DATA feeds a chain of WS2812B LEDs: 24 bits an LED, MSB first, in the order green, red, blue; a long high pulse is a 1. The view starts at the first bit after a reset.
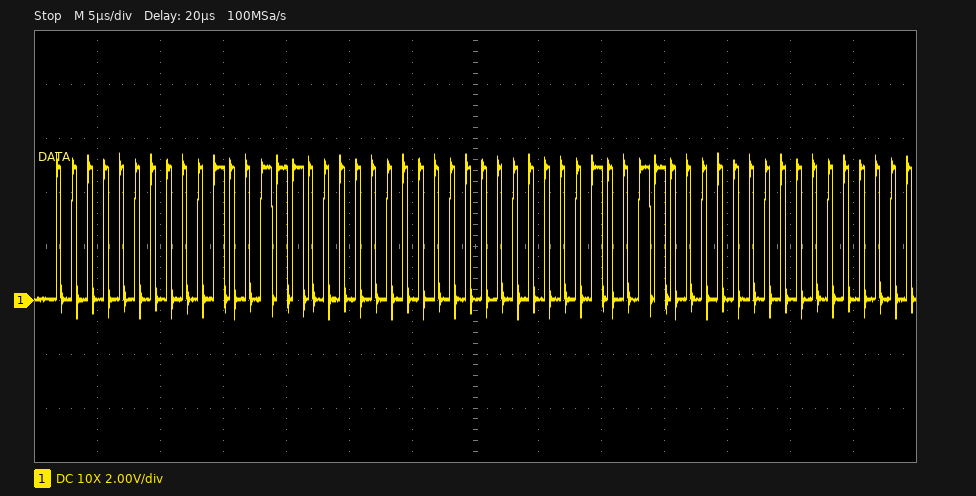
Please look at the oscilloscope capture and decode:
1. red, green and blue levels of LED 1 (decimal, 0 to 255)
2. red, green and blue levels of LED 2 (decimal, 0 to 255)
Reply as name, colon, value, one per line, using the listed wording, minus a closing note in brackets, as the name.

red, green and blue levels of LED 1: 39, 0, 0
red, green and blue levels of LED 2: 38, 0, 0
